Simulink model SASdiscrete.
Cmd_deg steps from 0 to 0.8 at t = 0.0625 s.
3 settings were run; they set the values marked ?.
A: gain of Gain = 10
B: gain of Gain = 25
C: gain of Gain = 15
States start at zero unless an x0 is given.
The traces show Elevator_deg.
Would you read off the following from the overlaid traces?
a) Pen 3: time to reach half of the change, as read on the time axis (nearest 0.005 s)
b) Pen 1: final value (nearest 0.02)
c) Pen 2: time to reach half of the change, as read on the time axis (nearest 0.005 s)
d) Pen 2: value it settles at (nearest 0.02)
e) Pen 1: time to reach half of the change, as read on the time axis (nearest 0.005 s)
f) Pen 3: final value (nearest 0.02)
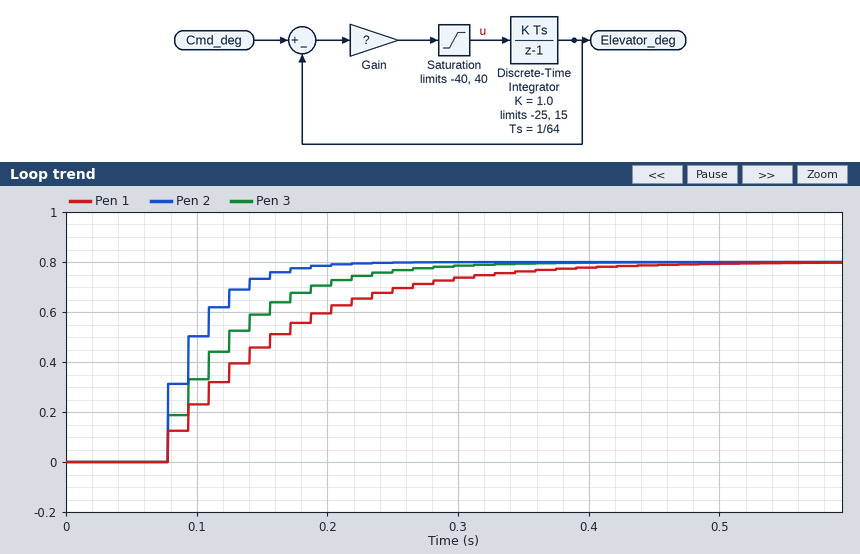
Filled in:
0.110 s
0.80
0.095 s
0.80
0.140 s
0.80
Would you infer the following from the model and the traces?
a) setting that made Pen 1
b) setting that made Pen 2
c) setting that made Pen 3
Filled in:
A
B
C
